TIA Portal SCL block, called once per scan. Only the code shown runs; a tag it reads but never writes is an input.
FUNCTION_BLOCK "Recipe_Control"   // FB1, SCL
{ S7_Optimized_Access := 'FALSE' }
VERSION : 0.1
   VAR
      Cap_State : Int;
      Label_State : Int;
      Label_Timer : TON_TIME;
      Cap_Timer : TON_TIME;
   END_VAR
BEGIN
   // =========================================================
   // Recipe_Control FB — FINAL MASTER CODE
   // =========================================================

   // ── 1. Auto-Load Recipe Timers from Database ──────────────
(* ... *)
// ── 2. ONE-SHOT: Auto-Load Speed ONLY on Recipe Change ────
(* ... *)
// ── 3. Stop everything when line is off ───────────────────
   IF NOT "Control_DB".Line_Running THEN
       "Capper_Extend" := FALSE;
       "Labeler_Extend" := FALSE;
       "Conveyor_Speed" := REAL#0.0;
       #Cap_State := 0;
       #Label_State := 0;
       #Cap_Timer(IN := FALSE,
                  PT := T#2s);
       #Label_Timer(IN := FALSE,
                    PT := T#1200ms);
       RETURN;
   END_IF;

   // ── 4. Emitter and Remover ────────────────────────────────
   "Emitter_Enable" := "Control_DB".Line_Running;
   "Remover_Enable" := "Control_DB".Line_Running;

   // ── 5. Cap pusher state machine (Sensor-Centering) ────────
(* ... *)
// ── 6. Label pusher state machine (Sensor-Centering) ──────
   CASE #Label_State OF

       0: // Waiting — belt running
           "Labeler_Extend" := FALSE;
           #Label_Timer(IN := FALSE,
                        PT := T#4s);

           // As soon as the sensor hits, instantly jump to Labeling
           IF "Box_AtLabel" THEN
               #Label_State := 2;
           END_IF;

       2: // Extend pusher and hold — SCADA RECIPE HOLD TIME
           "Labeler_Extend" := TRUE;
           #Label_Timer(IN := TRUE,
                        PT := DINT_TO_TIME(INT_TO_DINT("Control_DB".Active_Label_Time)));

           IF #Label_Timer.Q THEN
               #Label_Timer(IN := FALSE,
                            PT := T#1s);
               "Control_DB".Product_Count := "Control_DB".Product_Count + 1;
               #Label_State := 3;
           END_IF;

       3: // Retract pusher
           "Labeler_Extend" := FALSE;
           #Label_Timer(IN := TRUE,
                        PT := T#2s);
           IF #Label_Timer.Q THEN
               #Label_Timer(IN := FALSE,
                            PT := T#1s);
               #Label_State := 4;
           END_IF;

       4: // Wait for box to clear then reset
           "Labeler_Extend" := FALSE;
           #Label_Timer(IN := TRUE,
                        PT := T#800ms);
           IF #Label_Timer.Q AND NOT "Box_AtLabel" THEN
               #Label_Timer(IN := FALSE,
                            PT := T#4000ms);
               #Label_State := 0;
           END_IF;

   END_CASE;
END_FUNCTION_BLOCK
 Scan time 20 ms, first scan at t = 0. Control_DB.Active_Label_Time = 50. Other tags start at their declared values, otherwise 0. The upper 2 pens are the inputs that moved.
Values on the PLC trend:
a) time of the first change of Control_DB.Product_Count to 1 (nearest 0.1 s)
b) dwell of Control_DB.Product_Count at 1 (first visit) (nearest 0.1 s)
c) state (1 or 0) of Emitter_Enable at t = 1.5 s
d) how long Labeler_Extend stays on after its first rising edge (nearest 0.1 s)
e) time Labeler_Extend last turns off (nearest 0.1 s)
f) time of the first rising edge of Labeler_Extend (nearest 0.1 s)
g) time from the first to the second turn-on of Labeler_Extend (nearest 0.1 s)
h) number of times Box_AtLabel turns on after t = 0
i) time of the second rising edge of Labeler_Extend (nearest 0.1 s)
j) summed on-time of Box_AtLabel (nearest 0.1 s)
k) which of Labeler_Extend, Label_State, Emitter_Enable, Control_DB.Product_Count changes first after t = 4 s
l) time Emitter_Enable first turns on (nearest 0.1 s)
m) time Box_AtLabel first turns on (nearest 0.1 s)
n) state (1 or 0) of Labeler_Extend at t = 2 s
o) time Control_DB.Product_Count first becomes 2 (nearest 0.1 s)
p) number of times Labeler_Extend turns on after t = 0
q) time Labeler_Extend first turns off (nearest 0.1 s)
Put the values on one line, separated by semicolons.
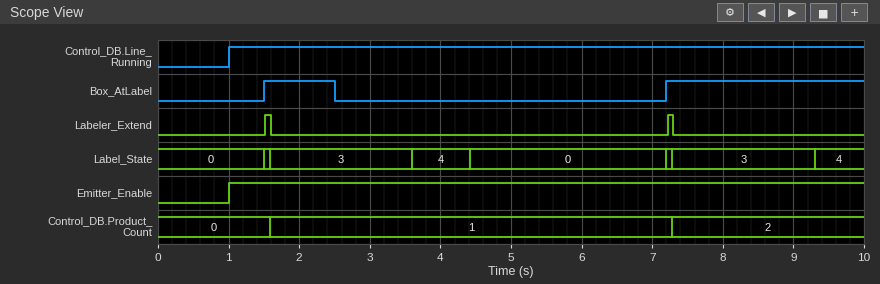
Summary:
1.6 s; 5.7 s; 1; 0.1 s; 7.3 s; 1.5 s; 5.7 s; 2; 7.2 s; 3.8 s; Label_State; 1.0 s; 1.5 s; 0; 7.3 s; 2; 1.6 s
